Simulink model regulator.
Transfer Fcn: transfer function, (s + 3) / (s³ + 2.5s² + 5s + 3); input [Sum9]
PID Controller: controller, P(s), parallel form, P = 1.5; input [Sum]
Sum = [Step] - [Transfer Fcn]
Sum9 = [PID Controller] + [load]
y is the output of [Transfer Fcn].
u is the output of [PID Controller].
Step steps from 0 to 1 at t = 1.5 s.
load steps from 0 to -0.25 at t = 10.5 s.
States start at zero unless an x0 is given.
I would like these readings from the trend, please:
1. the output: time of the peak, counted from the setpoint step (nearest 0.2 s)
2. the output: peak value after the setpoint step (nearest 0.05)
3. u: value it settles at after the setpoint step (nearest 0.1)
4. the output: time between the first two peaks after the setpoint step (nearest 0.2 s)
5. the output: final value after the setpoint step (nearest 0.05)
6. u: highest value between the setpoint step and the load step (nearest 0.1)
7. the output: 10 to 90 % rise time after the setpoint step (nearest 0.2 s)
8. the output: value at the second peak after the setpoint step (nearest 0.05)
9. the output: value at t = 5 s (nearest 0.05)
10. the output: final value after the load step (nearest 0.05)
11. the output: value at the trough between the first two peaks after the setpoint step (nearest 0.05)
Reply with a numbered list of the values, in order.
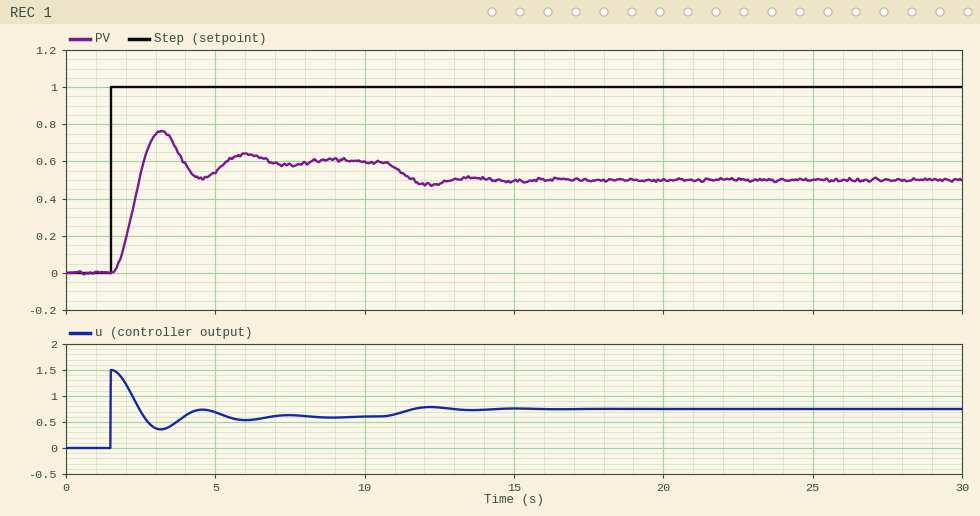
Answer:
1. 1.6 s
2. 0.75
3. 0.6
4. 2.8 s
5. 0.60
6. 1.5
7. 0.8 s
8. 0.65
9. 0.55
10. 0.50
11. 0.50
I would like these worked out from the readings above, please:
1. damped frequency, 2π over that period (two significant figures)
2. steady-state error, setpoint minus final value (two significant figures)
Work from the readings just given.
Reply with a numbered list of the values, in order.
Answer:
1. 2.2 rad/s
2. 0.40
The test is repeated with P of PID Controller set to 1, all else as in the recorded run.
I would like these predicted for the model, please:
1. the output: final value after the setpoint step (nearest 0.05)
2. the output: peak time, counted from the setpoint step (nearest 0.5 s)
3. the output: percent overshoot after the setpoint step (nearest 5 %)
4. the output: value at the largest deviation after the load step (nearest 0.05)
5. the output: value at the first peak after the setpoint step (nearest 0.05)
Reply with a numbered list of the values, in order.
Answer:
1. 0.50
2. 2.0 s
3. 20 %
4. 0.35
5. 0.60
